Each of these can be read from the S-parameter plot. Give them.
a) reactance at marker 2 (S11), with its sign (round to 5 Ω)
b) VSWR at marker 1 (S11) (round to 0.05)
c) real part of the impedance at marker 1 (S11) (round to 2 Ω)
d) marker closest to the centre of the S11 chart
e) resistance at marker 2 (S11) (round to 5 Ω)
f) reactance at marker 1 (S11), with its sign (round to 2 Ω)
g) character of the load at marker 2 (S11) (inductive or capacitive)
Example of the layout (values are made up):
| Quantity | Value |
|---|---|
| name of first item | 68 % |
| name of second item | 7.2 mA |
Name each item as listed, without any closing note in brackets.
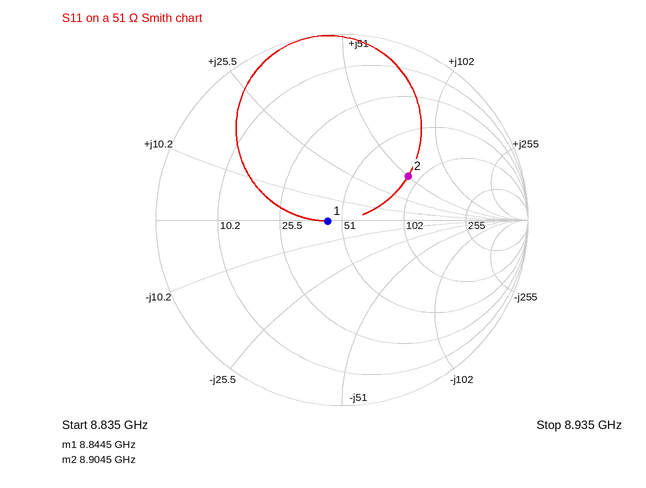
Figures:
| Quantity | Value |
|---|---|
| reactance at marker 2 (S11), with its sign | +50 Ω |
| VSWR at marker 1 (S11) | 1.15 |
| real part of the impedance at marker 1 (S11) | 44 Ω |
| marker closest to the centre of the S11 chart | marker 1 |
| resistance at marker 2 (S11) | 90 Ω |
| reactance at marker 1 (S11), with its sign | 0 Ω |
| character of the load at marker 2 (S11) | inductive |
